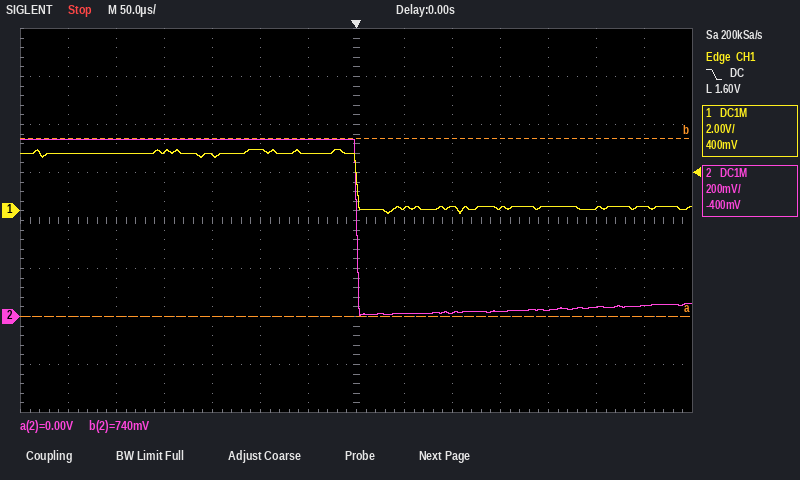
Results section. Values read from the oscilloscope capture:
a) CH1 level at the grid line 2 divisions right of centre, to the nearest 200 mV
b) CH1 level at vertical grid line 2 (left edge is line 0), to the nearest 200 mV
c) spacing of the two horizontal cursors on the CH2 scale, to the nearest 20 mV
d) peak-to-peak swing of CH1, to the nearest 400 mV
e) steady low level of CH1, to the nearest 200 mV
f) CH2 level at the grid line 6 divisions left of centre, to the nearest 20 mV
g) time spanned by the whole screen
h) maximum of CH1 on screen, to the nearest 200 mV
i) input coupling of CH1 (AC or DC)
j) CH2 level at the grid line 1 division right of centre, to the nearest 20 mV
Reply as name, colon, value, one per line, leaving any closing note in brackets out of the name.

CH1 level at the grid line 2 divisions right of centre, to the nearest 200 mV: 200 mV
CH1 level at vertical grid line 2 (left edge is line 0), to the nearest 200 mV: 2.4 V
spacing of the two horizontal cursors on the CH2 scale, to the nearest 20 mV: 740 mV
peak-to-peak swing of CH1, to the nearest 400 mV: 2.8 V
steady low level of CH1, to the nearest 200 mV: 200 mV
CH2 level at the grid line 6 divisions left of centre, to the nearest 20 mV: 740 mV
time spanned by the whole screen: 700 µs
maximum of CH1 on screen, to the nearest 200 mV: 2.6 V
input coupling of CH1: DC
CH2 level at the grid line 1 division right of centre, to the nearest 20 mV: 20 mV
